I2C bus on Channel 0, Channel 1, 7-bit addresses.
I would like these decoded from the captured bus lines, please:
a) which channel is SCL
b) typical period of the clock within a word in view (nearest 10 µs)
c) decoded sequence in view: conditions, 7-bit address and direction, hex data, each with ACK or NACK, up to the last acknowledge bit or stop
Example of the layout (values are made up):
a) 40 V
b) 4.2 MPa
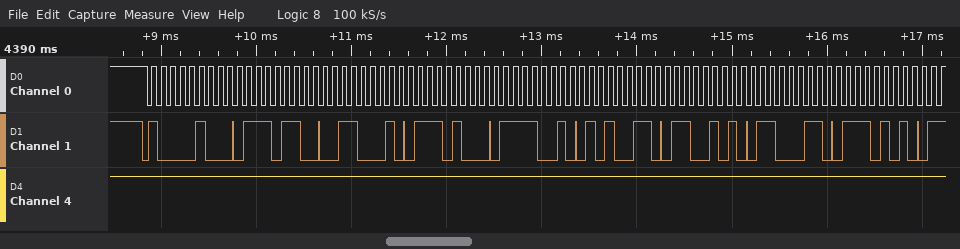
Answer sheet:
a) Channel 0
b) 100 µs
c) start, address 42 write ACK, 76 ACK, 31 ACK, 74 ACK, 79 ACK, 53 ACK, 65 ACK, 63 ACK, 75 ACK
